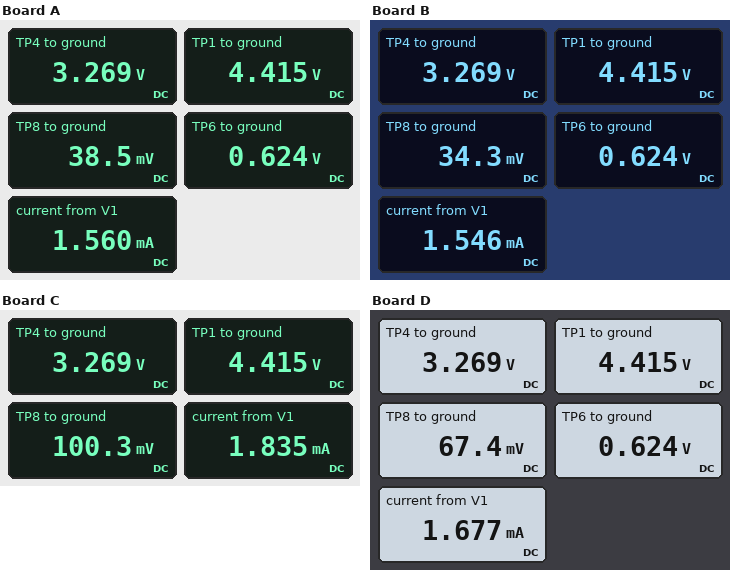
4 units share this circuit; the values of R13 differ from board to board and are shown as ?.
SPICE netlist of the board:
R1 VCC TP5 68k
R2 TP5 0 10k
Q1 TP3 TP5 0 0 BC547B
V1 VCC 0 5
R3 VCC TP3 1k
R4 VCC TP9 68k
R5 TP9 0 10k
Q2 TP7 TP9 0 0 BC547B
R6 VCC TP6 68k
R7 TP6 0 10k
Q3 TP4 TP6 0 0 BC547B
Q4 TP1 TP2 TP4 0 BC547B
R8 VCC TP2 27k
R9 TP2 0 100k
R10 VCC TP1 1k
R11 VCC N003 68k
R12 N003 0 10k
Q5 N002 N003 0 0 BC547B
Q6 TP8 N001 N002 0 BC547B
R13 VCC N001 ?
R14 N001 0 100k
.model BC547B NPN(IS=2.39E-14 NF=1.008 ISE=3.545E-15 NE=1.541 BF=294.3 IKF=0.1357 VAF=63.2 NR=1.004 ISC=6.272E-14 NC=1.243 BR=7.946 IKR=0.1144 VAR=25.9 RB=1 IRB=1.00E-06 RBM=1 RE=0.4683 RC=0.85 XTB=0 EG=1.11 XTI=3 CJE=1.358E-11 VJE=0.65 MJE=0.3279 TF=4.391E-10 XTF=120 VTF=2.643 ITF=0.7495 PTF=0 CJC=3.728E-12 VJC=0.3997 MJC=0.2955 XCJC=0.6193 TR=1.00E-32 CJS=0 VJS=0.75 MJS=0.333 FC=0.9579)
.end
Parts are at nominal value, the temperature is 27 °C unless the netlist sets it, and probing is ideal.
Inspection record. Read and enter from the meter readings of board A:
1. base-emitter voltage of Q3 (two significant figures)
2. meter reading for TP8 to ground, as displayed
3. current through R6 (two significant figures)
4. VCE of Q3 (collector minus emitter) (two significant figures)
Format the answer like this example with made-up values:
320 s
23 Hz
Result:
620 mV
38.5 mV
64 µA
3.3 V
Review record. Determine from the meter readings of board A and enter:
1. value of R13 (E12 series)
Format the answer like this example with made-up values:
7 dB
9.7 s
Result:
56 kΩ
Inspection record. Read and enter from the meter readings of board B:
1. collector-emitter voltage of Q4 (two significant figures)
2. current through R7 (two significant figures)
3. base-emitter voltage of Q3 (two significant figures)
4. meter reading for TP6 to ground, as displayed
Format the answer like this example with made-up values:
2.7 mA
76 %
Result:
1.1 V
62 µA
620 mV
0.624 V
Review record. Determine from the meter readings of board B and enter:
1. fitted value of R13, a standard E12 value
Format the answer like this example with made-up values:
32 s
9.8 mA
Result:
68 kΩ
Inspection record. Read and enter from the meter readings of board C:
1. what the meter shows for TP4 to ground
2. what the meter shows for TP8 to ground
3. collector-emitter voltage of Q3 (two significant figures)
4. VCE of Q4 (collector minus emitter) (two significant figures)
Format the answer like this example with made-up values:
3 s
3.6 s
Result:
3.269 V
100.3 mV
3.3 V
1.1 V
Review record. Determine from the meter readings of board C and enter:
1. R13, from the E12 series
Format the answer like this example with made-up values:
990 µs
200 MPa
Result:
12 kΩ
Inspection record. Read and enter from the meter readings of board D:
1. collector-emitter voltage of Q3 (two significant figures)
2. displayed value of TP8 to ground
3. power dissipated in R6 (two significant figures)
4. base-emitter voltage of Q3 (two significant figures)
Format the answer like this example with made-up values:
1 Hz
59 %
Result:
3.3 V
67.4 mV
280 µW
620 mV
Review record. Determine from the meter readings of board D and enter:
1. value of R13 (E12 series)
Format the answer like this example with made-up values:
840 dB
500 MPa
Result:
22 kΩ
